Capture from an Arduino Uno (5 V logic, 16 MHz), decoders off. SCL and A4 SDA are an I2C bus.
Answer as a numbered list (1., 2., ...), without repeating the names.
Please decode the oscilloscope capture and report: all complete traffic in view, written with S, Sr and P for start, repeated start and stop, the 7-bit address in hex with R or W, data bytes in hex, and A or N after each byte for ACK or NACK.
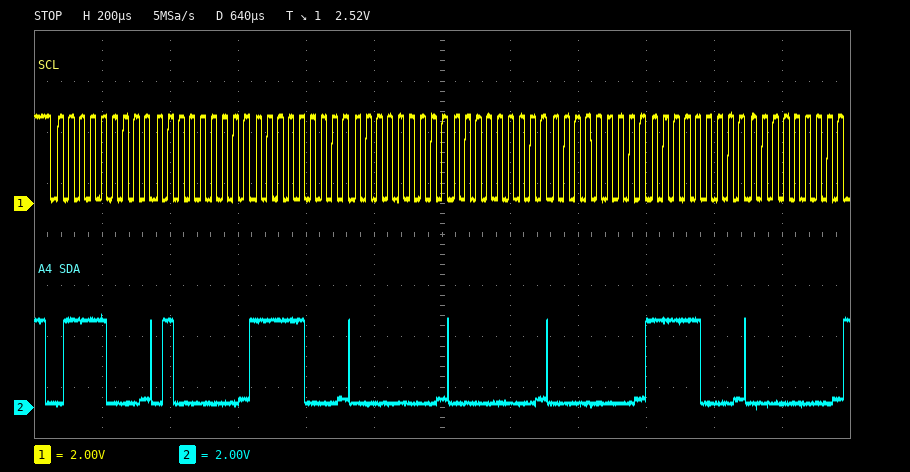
1. S 3CW A 40 A F8 A 00 A 00 A 00 A F8 A 00 A
